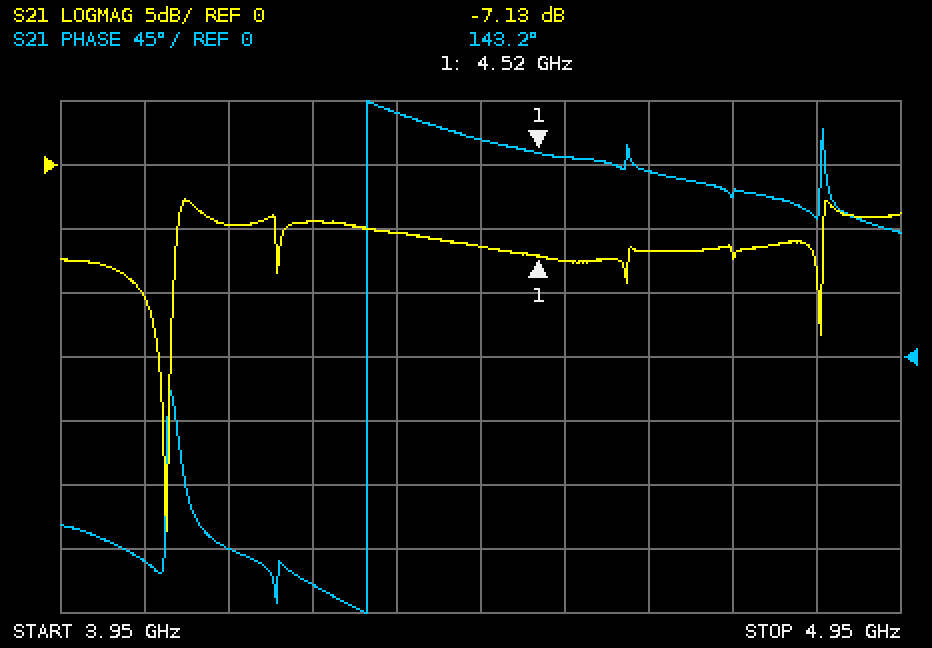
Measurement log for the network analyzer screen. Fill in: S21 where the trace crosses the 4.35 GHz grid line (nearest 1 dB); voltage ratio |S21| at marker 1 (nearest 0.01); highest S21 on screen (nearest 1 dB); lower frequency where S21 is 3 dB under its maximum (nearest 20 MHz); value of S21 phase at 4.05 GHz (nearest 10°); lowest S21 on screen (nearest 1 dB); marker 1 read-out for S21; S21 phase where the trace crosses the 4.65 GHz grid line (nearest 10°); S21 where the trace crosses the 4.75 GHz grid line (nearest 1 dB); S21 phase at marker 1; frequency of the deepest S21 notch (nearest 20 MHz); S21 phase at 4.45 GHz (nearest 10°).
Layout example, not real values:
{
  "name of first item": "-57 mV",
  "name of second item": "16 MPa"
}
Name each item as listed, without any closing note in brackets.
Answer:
{
  "S21 where the trace crosses the 4.35 GHz grid line": "-5 dB",
  "voltage ratio |S21| at marker 1": "0.44",
  "highest S21 on screen": "-3 dB",
  "lower frequency where S21 is 3 dB under its maximum": "4.08 GHz",
  "value of S21 phase at 4.05 GHz": "-140°",
  "lowest S21 on screen": "-29 dB",
  "marker 1 read-out for S21": "-7.13 dB",
  "S21 phase where the trace crosses the 4.65 GHz grid line": "130°",
  "S21 where the trace crosses the 4.75 GHz grid line": "-7 dB",
  "S21 phase at marker 1": "143.2°",
  "frequency of the deepest S21 notch": "4.08 GHz",
  "S21 phase at 4.45 GHz": "150°"
}
